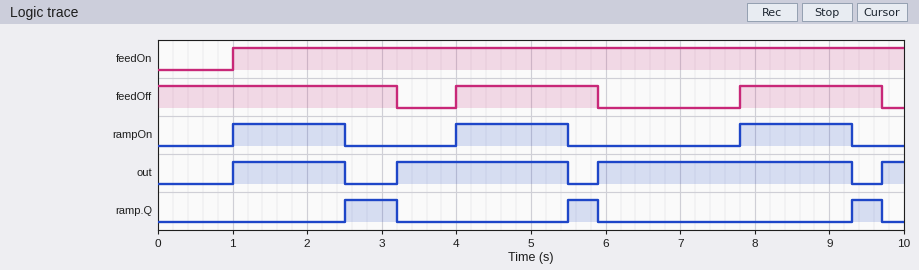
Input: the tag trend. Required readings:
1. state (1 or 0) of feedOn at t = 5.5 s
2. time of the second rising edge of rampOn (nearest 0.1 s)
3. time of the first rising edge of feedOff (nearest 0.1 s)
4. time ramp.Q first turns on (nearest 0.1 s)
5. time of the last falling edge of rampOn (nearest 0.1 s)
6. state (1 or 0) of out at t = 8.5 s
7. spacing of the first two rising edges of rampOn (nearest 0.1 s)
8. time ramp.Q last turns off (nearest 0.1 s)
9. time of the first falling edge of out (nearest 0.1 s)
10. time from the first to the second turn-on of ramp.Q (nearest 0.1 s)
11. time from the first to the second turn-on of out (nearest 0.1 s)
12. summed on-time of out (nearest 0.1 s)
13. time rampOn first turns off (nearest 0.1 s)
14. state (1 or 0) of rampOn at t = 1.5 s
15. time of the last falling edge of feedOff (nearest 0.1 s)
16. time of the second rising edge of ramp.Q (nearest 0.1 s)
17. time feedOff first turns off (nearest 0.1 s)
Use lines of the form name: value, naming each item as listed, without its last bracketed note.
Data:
state (1 or 0) of feedOn at t = 5.5 s: 1
time of the second rising edge of rampOn: 4.0 s
time of the first rising edge of feedOff: 4.0 s
time ramp.Q first turns on: 2.5 s
time of the last falling edge of rampOn: 9.3 s
state (1 or 0) of out at t = 8.5 s: 1
spacing of the first two rising edges of rampOn: 3.0 s
time ramp.Q last turns off: 9.7 s
time of the first falling edge of out: 2.5 s
time from the first to the second turn-on of ramp.Q: 3.0 s
time from the first to the second turn-on of out: 2.2 s
summed on-time of out: 7.5 s
time rampOn first turns off: 2.5 s
state (1 or 0) of rampOn at t = 1.5 s: 1
time of the last falling edge of feedOff: 9.7 s
time of the second rising edge of ramp.Q: 5.5 s
time feedOff first turns off: 3.2 s
